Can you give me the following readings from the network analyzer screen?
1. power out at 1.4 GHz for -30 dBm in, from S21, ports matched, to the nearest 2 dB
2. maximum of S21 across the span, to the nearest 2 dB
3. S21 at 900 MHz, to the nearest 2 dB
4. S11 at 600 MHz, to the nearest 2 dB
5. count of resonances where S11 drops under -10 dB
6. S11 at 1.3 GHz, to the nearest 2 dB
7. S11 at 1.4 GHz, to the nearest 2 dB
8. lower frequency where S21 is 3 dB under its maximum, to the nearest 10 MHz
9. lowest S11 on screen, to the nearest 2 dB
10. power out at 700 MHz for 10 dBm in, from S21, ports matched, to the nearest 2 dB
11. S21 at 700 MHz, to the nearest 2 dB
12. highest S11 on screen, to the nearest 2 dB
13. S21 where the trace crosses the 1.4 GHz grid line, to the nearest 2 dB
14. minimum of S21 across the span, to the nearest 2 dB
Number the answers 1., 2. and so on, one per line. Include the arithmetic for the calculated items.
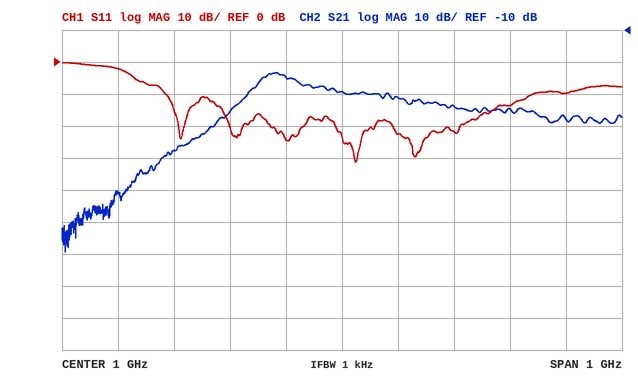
1. -30 dBm + (-38 dB) = -68 dBm
2. -24 dB
3. -24 dB
4. -2 dB
5. 5
6. -14 dB
7. -10 dB
8. 850 MHz
9. -32 dB
10. 10 dBm + (-48 dB) = -38 dBm
11. -48 dB
12. 0 dB
13. -38 dB
14. -80 dB
